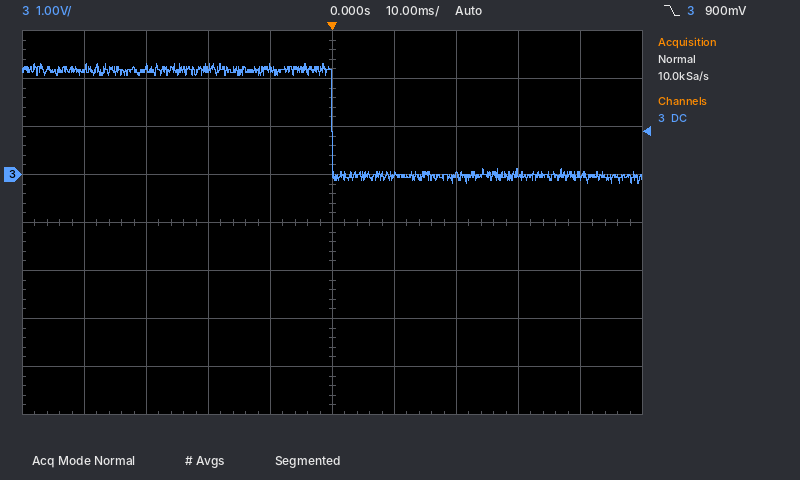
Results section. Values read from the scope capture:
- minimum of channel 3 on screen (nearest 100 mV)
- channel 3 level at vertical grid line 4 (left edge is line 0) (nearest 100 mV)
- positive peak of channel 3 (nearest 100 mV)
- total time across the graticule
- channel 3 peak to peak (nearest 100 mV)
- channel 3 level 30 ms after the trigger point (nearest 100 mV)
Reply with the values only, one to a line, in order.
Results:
-200 mV
2.2 V
2.3 V
100 ms
2.5 V
0.0 V
